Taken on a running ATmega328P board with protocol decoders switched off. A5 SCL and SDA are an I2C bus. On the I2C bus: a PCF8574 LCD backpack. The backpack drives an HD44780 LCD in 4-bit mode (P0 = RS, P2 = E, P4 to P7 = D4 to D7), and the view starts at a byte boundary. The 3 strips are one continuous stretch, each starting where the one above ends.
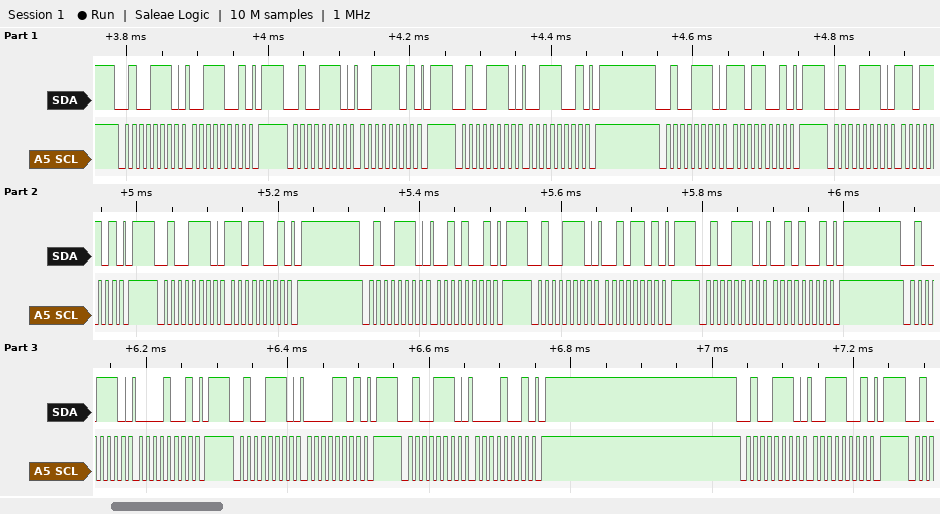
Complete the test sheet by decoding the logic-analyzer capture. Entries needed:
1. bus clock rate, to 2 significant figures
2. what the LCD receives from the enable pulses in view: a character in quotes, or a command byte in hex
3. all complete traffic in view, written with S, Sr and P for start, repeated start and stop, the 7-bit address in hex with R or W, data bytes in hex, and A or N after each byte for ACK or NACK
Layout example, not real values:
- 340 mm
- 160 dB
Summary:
- 100 kHz
- '=' ' '
- S 27W A 39 A P S 27W A 3D A P S 27W A 39 A P S 27W A D9 A P S 27W A DD A P S 27W A D9 A P S 27W A 29 A P S 27W A 2D A P S 27W A 29 A P S 27W A 09 A P S 27W A 0D A P S 27W A 09 A P S 27W A 39 A P
